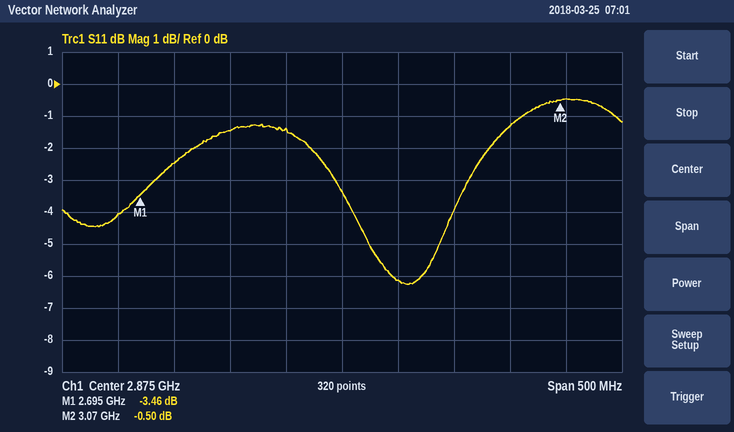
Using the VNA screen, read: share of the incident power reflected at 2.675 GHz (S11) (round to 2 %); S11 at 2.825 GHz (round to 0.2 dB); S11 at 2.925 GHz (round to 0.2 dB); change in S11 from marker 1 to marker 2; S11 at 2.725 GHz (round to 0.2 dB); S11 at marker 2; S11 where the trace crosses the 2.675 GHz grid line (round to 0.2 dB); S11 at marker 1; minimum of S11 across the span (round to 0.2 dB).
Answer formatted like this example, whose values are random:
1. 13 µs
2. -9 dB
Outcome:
1. 40 %
2. -1.4 dB
3. -6.2 dB
4. 2.96 dB
5. -2.4 dB
6. -0.50 dB
7. -4.0 dB
8. -3.46 dB
9. -6.2 dB
